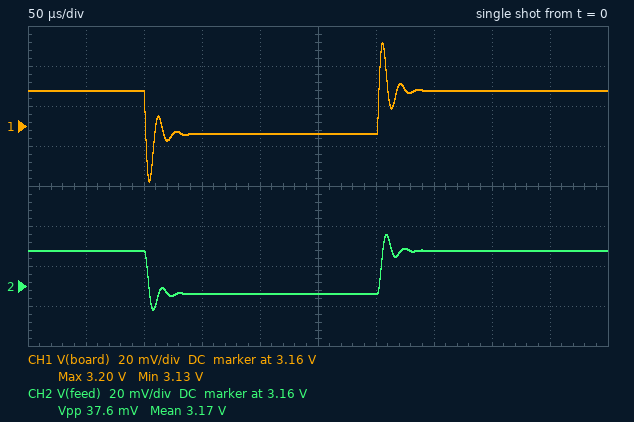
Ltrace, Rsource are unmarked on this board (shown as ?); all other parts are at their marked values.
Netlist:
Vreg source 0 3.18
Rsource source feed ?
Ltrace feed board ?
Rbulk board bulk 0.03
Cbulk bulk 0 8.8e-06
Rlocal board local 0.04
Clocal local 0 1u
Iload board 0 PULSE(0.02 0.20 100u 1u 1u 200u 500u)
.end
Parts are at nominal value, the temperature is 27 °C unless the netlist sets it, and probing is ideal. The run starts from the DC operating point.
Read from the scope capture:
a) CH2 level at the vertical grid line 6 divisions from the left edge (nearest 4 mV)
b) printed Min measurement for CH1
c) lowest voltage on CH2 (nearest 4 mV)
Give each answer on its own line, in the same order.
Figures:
3.156 V
3.13 V
3.148 V
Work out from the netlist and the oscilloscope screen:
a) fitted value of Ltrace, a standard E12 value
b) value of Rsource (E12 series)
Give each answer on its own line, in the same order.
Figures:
560 nH
0.12 Ω
